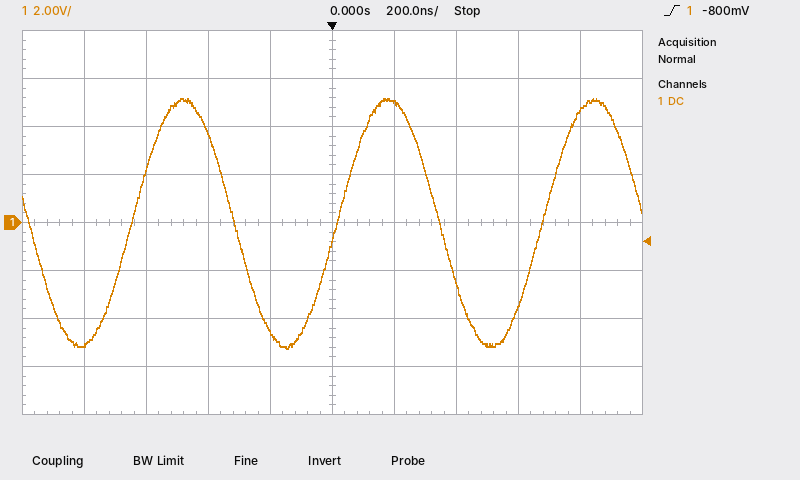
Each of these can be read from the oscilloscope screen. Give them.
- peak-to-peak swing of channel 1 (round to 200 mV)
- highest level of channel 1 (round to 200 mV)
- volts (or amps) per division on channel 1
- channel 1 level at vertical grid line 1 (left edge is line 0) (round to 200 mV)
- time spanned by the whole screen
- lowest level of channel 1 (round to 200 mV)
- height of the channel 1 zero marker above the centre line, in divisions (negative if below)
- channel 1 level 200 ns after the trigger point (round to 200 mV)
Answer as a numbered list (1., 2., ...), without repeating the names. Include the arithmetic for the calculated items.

1. 5.2 V − (-5.2 V) = 10.4 V
2. 5.2 V
3. 2 V
4. -5.0 V
5. 2 µs
6. -5.2 V
7. 0.0 div
8. 5.0 V
